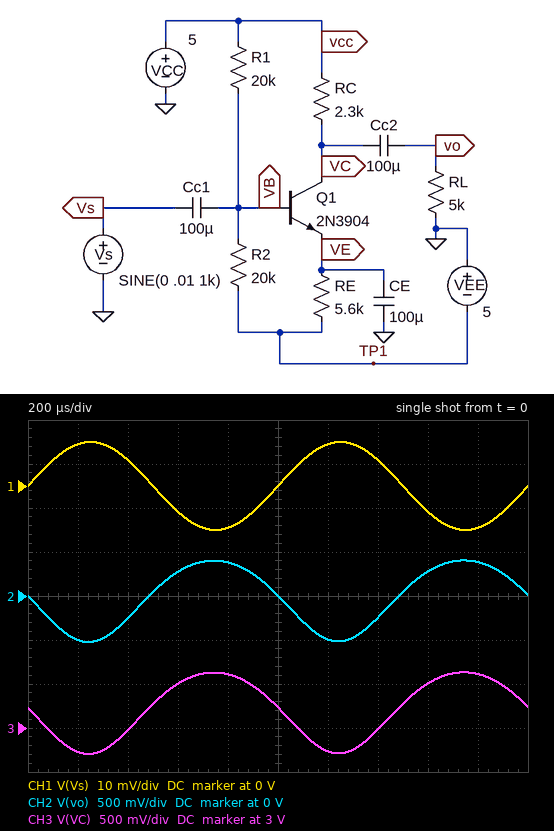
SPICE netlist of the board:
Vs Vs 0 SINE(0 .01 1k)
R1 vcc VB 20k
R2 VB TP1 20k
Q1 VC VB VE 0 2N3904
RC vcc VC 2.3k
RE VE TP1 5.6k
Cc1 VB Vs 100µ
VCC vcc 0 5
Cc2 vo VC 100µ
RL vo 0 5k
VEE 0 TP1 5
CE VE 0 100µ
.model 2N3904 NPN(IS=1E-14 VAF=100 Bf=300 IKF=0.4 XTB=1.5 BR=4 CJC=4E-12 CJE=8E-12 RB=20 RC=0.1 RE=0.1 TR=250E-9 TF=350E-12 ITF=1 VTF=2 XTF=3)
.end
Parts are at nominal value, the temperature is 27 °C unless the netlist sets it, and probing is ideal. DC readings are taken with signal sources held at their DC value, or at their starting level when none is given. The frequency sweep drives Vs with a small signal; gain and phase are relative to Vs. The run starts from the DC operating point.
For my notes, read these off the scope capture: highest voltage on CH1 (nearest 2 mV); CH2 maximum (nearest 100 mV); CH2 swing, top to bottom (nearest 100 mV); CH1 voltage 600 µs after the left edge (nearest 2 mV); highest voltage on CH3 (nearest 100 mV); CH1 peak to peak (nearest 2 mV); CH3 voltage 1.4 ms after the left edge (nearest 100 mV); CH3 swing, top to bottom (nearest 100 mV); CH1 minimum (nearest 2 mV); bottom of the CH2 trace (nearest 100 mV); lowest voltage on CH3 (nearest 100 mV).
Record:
10 mV
400 mV
900 mV
-6 mV
3.6 V
20 mV
3.0 V
900 mV
-10 mV
-500 mV
2.7 V
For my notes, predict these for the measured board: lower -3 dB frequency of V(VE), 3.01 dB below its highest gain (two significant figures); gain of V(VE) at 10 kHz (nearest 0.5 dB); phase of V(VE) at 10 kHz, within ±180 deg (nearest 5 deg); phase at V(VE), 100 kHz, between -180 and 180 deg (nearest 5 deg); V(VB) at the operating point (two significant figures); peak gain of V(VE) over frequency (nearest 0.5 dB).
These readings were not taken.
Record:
160 mHz
-46.5 dB
-90 deg
-90 deg
-25 mV
0 dB
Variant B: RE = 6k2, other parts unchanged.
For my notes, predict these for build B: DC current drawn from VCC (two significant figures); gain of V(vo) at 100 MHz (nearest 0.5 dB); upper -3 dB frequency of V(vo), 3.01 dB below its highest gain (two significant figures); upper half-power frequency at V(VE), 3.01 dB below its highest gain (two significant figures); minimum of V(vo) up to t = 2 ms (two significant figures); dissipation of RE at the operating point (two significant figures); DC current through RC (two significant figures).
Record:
950 µA
21.0 dB
28 MHz
43 Hz
-480 mV
3.0 mW
700 µA
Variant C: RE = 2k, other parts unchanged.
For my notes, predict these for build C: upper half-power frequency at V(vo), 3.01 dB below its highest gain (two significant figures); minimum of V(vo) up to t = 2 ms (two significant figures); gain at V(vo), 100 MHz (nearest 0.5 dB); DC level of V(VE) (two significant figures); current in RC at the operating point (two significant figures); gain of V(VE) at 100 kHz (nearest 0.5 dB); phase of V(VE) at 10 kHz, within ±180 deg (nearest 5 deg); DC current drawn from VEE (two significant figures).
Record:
10 MHz
-800 mV
22.0 dB
-750 mV
2.1 mA
-58.0 dB
-90 deg
2.4 mA
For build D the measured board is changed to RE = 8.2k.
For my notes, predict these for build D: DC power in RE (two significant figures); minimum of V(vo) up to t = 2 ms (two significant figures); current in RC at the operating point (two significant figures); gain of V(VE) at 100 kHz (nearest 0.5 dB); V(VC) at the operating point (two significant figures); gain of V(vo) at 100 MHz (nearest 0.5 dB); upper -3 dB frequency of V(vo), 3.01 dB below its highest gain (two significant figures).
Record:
2.3 mW
-370 mV
530 µA
-70.0 dB
3.8 V
19.5 dB
32 MHz
